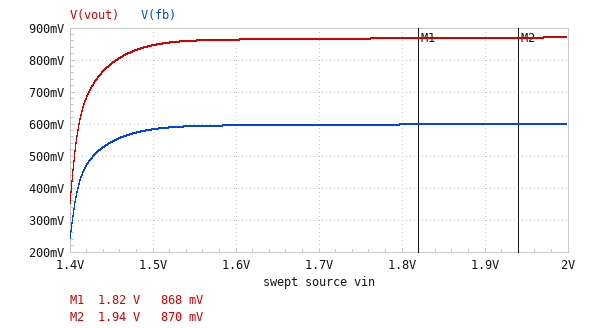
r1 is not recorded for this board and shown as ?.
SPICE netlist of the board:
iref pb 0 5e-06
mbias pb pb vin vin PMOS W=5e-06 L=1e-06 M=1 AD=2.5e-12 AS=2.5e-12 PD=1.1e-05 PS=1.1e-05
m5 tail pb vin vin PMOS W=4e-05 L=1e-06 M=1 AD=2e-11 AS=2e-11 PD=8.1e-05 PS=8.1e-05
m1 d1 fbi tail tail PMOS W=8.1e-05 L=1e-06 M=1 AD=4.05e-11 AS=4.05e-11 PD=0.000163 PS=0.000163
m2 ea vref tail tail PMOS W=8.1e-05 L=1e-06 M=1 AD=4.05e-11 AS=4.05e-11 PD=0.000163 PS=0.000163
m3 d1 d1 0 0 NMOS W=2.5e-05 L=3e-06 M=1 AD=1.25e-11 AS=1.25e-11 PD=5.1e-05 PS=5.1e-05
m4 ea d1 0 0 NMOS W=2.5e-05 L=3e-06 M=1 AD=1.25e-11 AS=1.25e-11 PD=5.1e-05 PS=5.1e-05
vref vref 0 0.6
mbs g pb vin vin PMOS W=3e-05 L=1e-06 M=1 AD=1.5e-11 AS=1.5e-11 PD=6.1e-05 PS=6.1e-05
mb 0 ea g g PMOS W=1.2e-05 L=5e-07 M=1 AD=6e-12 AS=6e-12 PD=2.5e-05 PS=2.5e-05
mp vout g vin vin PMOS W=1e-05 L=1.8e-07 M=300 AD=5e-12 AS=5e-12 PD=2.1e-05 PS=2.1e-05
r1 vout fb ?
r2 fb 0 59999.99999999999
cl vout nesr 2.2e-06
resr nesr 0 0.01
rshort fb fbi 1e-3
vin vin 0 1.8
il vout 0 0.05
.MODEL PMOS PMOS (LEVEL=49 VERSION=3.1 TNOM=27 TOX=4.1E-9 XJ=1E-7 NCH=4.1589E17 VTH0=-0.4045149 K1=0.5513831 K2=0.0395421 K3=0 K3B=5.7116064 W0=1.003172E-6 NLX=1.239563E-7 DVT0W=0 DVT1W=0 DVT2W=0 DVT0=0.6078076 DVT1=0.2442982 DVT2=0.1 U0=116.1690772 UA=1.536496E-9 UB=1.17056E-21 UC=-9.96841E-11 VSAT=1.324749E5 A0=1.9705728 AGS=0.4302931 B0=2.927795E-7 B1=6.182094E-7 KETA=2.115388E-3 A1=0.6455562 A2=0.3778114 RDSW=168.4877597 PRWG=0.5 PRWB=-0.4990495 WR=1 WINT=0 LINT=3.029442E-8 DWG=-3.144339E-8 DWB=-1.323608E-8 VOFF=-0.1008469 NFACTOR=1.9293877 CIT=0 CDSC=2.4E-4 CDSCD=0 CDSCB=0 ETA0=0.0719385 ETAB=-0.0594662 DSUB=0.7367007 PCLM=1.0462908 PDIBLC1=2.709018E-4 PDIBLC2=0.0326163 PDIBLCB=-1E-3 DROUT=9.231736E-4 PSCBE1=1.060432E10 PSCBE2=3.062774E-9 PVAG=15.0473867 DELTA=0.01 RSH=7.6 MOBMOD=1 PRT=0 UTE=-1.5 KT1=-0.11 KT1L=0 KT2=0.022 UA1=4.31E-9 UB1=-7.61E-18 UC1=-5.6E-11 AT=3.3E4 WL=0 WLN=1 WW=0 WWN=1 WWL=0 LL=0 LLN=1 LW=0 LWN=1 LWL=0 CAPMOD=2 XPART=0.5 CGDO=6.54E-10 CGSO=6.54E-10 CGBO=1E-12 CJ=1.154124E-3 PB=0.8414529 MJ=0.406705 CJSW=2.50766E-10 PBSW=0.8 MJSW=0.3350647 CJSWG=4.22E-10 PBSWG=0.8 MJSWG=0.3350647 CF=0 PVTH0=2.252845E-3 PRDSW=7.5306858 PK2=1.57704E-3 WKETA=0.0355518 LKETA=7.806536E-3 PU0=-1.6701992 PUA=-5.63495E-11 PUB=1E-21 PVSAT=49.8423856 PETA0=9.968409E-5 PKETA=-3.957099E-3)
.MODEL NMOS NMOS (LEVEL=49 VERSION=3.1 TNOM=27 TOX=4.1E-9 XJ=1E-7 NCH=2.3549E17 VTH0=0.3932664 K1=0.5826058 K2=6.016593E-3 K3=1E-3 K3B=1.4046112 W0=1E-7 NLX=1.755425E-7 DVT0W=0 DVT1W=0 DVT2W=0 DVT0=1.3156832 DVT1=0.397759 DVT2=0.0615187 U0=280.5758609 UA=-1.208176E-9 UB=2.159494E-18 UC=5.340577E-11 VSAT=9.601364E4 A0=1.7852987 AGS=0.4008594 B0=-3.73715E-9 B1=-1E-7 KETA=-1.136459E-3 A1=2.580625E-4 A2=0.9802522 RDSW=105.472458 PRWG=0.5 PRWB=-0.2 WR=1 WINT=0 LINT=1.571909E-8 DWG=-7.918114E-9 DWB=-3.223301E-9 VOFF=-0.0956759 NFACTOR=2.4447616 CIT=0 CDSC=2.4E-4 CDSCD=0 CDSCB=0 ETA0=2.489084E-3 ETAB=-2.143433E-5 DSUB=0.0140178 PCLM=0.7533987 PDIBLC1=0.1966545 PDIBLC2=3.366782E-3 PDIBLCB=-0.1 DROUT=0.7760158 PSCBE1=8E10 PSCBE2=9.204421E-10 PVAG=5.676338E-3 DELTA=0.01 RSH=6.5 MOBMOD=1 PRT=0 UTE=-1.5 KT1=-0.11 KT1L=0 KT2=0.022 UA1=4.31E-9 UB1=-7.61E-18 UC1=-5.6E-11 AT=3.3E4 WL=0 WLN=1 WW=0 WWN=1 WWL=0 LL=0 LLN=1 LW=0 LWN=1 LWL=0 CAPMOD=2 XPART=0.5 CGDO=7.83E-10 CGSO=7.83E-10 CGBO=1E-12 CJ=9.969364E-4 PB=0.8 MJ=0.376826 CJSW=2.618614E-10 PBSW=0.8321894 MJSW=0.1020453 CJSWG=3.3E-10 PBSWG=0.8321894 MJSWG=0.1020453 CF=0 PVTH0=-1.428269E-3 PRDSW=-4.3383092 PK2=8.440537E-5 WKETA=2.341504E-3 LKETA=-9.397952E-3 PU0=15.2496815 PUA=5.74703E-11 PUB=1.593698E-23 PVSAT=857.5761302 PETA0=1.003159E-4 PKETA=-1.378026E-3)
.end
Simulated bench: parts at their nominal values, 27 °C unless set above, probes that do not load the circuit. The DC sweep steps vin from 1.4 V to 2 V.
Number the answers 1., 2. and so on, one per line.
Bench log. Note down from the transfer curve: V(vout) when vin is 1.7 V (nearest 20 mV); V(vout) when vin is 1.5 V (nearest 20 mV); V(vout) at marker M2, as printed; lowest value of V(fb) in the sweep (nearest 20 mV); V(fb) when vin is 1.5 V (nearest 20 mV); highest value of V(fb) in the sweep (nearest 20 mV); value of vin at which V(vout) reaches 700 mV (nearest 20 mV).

1. 860 mV
2. 840 mV
3. 870 mV
4. 240 mV
5. 580 mV
6. 600 mV
7. 1.42 V
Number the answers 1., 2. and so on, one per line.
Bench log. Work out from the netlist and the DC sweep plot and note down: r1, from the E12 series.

1. 27 kΩ
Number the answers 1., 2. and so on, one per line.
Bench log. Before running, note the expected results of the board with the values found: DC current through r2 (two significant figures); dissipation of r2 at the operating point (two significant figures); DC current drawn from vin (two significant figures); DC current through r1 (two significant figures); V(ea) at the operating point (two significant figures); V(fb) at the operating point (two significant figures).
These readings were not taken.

1. 10 µA
2. 6.0 µW
3. 50 mA
4. 10 µA
5. 400 mV
6. 600 mV
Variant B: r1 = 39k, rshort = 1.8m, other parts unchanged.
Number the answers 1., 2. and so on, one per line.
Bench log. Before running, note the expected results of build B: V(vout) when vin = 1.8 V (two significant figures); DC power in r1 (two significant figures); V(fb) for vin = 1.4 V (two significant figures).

1. 990 mV
2. 3.9 µW
3. 210 mV
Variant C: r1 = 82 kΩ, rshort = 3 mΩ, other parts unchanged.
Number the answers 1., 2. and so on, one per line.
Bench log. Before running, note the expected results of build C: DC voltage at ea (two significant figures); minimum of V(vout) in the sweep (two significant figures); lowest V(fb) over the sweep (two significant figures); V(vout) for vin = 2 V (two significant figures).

1. 380 mV
2. 350 mV
3. 150 mV
4. 1.4 V
